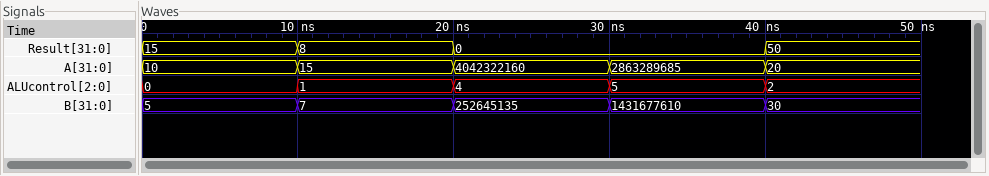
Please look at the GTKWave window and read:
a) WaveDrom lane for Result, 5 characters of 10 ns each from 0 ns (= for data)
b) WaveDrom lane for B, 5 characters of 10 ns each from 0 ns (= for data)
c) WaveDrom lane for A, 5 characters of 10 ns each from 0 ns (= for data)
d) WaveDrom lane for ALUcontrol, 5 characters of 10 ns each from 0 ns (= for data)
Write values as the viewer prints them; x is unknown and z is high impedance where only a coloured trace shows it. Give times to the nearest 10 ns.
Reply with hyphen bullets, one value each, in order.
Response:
- {name: 'Result', wave: '===.=', data: '15 8 0 50'}
- {name: 'B', wave: '=====', data: '5 7 252645135 1431677610 30'}
- {name: 'A', wave: '=====', data: '10 15 4042322160 2863289685 20'}
- {name: 'ALUcontrol', wave: '=====', data: '0 1 4 5 2'}
